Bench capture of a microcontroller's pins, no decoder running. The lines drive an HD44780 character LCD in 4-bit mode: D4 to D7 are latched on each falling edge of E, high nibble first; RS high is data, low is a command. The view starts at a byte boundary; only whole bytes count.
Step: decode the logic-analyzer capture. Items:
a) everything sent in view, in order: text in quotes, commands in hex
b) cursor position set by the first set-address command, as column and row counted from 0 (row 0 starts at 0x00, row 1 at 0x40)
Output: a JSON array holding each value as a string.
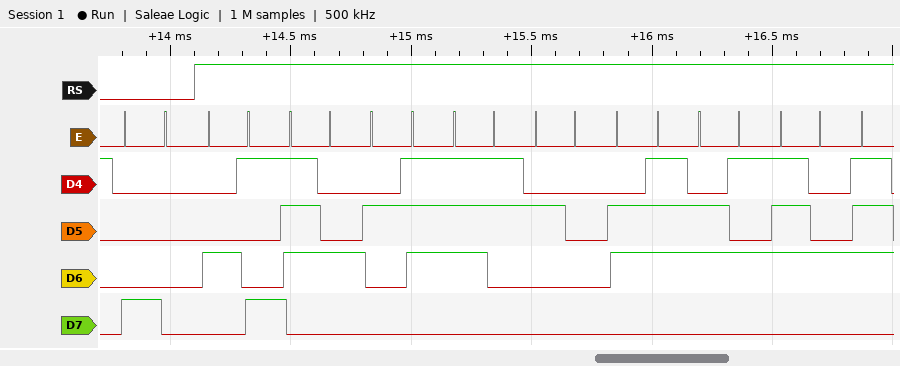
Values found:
["0x80 \"It's get\"", "column 0, row 0"]
